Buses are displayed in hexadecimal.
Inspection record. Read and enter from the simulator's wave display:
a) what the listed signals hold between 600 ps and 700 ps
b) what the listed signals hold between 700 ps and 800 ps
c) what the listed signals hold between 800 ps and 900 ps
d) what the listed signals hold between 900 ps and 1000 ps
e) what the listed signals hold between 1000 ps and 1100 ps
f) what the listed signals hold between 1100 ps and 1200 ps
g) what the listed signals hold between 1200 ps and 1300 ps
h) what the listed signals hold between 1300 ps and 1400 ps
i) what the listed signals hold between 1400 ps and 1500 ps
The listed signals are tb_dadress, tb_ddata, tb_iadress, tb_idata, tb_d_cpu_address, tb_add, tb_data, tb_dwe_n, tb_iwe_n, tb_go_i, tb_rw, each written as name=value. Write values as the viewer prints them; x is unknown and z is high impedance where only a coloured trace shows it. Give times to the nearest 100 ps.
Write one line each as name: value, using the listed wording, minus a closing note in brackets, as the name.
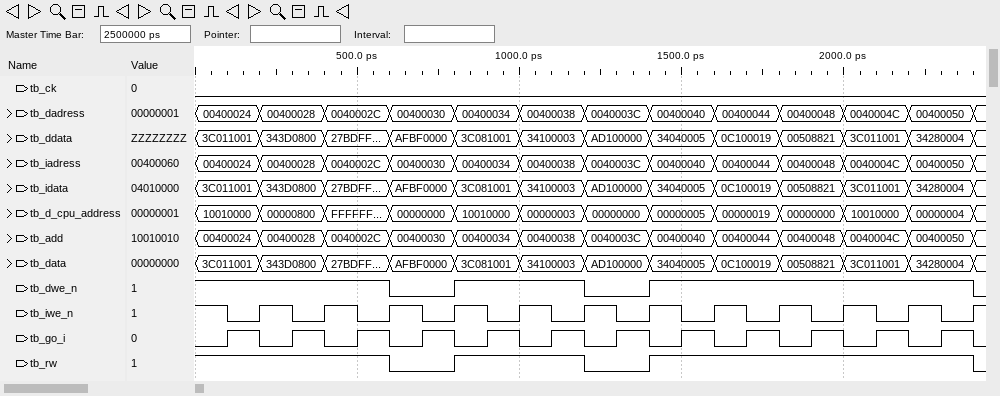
what the listed signals hold between 600 ps and 700 ps: tb_dadress=00400030, tb_ddata=AFBF0000, tb_iadress=00400030, tb_idata=AFBF0000, tb_d_cpu_address=00000000, tb_add=00400030, tb_data=AFBF0000, tb_dwe_n=0, tb_iwe_n=1, tb_go_i=0, tb_rw=0
what the listed signals hold between 700 ps and 800 ps: tb_dadress=00400030, tb_ddata=AFBF0000, tb_iadress=00400030, tb_idata=AFBF0000, tb_d_cpu_address=00000000, tb_add=00400030, tb_data=AFBF0000, tb_dwe_n=0, tb_iwe_n=0, tb_go_i=1, tb_rw=0
what the listed signals hold between 800 ps and 900 ps: tb_dadress=00400034, tb_ddata=3C081001, tb_iadress=00400034, tb_idata=3C081001, tb_d_cpu_address=10010000, tb_add=00400034, tb_data=3C081001, tb_dwe_n=1, tb_iwe_n=1, tb_go_i=0, tb_rw=1
what the listed signals hold between 900 ps and 1000 ps: tb_dadress=00400034, tb_ddata=3C081001, tb_iadress=00400034, tb_idata=3C081001, tb_d_cpu_address=10010000, tb_add=00400034, tb_data=3C081001, tb_dwe_n=1, tb_iwe_n=0, tb_go_i=1, tb_rw=1
what the listed signals hold between 1000 ps and 1100 ps: tb_dadress=00400038, tb_ddata=34100003, tb_iadress=00400038, tb_idata=34100003, tb_d_cpu_address=00000003, tb_add=00400038, tb_data=34100003, tb_dwe_n=1, tb_iwe_n=1, tb_go_i=0, tb_rw=1
what the listed signals hold between 1100 ps and 1200 ps: tb_dadress=00400038, tb_ddata=34100003, tb_iadress=00400038, tb_idata=34100003, tb_d_cpu_address=00000003, tb_add=00400038, tb_data=34100003, tb_dwe_n=1, tb_iwe_n=0, tb_go_i=1, tb_rw=1
what the listed signals hold between 1200 ps and 1300 ps: tb_dadress=0040003C, tb_ddata=AD100000, tb_iadress=0040003C, tb_idata=AD100000, tb_d_cpu_address=00000000, tb_add=0040003C, tb_data=AD100000, tb_dwe_n=0, tb_iwe_n=1, tb_go_i=0, tb_rw=0
what the listed signals hold between 1300 ps and 1400 ps: tb_dadress=0040003C, tb_ddata=AD100000, tb_iadress=0040003C, tb_idata=AD100000, tb_d_cpu_address=00000000, tb_add=0040003C, tb_data=AD100000, tb_dwe_n=0, tb_iwe_n=0, tb_go_i=1, tb_rw=0
what the listed signals hold between 1400 ps and 1500 ps: tb_dadress=00400040, tb_ddata=34040005, tb_iadress=00400040, tb_idata=34040005, tb_d_cpu_address=00000005, tb_add=00400040, tb_data=34040005, tb_dwe_n=1, tb_iwe_n=1, tb_go_i=0, tb_rw=1
